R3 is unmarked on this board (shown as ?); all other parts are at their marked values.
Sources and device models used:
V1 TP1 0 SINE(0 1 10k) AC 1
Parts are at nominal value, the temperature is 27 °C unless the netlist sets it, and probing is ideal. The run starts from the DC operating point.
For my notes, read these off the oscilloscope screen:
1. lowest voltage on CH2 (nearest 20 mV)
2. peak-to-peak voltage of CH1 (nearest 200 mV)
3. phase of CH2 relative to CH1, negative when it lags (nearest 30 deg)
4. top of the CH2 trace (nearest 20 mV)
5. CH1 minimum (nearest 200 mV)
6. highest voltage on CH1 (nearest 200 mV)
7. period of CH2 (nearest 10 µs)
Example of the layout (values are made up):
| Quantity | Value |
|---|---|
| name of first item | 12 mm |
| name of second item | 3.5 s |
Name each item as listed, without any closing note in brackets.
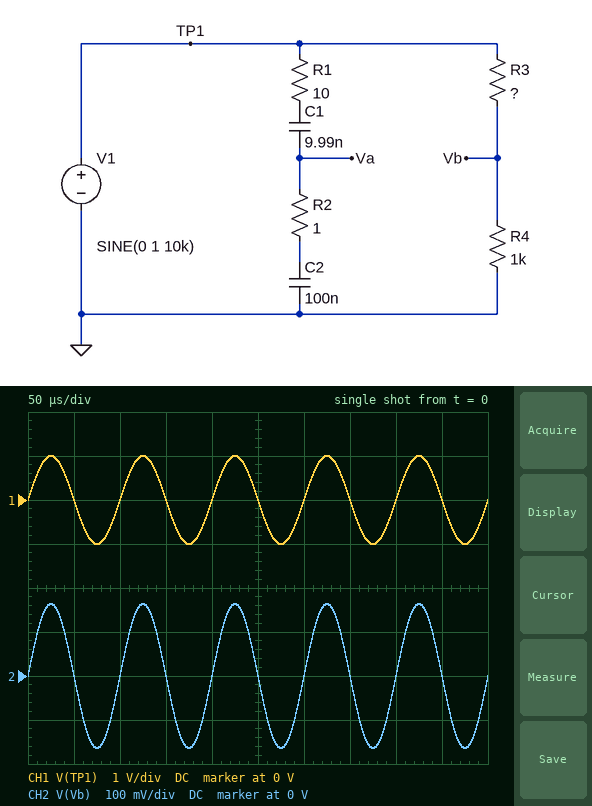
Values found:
| Quantity | Value |
|---|---|
| lowest voltage on CH2 | -160 mV |
| peak-to-peak voltage of CH1 | 2.0 V |
| phase of CH2 relative to CH1, negative when it lags | 0 deg |
| top of the CH2 trace | 160 mV |
| CH1 minimum | -1.0 V |
| highest voltage on CH1 | 1.0 V |
| period of CH2 | 100 µs |
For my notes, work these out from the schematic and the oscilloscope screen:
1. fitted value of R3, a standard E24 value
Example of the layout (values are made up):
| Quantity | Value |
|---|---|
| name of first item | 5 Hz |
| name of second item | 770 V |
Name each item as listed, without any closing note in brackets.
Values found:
| Quantity | Value |
|---|---|
| fitted value of R3, a standard E24 value | 5.1 kΩ |
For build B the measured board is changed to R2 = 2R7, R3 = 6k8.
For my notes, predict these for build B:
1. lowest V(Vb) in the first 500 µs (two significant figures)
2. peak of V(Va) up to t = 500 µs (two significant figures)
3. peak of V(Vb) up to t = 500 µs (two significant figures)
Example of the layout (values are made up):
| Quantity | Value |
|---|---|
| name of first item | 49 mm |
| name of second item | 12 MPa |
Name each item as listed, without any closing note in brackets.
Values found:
| Quantity | Value |
|---|---|
| lowest V(Vb) in the first 500 µs | -130 mV |
| peak of V(Va) up to t = 500 µs | 91 mV |
| peak of V(Vb) up to t = 500 µs | 130 mV |
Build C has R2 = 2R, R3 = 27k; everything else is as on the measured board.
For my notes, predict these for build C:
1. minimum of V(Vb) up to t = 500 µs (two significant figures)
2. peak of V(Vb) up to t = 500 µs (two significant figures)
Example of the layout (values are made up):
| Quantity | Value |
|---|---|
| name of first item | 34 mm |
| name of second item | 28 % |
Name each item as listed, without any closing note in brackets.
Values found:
| Quantity | Value |
|---|---|
| minimum of V(Vb) up to t = 500 µs | -36 mV |
| peak of V(Vb) up to t = 500 µs | 36 mV |
